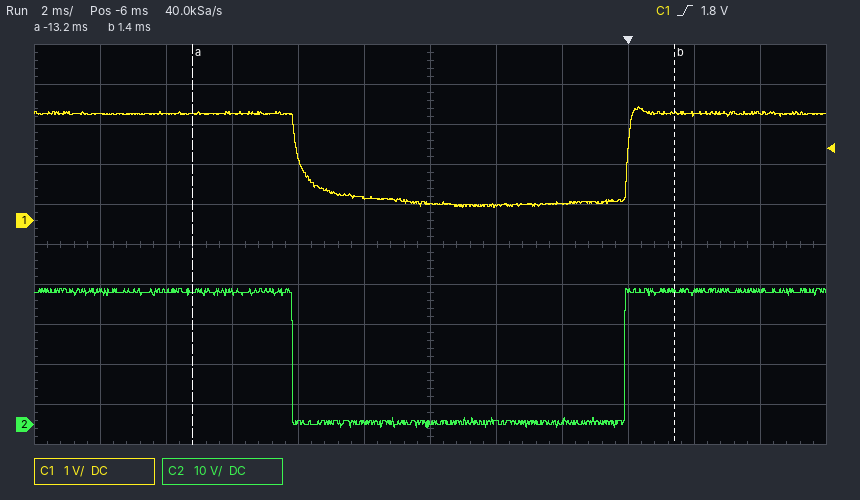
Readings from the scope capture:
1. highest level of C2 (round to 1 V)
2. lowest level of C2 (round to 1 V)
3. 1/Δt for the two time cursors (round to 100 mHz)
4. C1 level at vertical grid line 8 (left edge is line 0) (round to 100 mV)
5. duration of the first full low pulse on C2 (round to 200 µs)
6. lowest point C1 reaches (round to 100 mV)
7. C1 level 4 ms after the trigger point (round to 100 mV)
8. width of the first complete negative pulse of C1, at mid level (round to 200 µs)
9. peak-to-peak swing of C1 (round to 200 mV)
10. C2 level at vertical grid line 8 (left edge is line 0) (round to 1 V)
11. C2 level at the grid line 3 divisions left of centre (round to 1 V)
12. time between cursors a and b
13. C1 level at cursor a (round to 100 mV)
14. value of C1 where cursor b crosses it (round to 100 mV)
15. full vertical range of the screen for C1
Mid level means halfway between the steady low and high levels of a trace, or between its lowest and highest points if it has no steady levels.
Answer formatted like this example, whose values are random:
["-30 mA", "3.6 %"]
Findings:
["34 V", "-1 V", "68.5 Hz", "400 mV", "10.0 ms", "300 mV", "2.7 V", "10.0 ms", "2.6 V", "1 V", "33 V", "14.6 ms", "2.7 V", "2.7 V", "10 V"]
